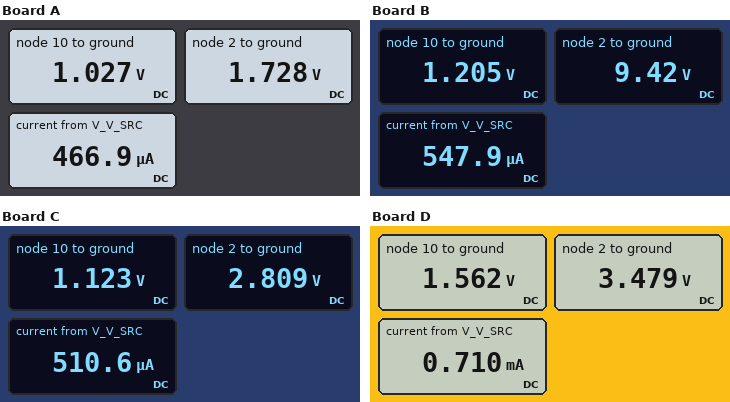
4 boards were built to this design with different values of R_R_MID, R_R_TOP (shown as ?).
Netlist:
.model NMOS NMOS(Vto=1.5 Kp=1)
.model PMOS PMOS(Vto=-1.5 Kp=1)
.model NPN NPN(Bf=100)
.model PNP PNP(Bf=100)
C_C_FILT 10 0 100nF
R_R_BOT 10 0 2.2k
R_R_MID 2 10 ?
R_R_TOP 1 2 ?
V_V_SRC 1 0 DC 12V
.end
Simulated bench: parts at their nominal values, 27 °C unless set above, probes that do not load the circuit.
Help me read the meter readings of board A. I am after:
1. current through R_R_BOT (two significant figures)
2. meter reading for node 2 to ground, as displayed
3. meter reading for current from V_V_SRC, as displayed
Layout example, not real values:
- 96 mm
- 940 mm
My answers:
- 470 µA
- 1.728 V
- 466.9 µA
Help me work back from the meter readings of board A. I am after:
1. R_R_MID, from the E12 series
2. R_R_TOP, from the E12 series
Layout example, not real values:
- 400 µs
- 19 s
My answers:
- 1.5 kΩ
- 22 kΩ
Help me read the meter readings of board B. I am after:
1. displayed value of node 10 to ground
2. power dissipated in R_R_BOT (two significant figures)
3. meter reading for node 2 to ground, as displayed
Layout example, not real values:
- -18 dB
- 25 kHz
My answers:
- 1.205 V
- 660 µW
- 9.42 V
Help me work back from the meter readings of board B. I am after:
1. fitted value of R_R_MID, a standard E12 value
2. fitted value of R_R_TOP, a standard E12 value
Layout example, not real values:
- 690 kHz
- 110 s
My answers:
- 15 kΩ
- 4.7 kΩ
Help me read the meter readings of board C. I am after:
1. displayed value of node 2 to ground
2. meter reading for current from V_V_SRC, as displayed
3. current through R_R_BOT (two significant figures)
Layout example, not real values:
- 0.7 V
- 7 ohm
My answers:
- 2.809 V
- 510.6 µA
- 510 µA
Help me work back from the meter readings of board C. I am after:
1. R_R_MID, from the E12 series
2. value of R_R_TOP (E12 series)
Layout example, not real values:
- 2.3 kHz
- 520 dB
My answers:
- 3.3 kΩ
- 18 kΩ
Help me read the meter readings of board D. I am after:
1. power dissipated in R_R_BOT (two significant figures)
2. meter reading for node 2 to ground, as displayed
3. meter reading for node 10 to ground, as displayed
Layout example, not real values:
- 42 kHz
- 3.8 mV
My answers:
- 1.1 mW
- 3.479 V
- 1.562 V
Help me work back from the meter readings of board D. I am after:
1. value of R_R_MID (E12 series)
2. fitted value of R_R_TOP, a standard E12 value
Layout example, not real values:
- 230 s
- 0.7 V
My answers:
- 2.7 kΩ
- 12 kΩ
